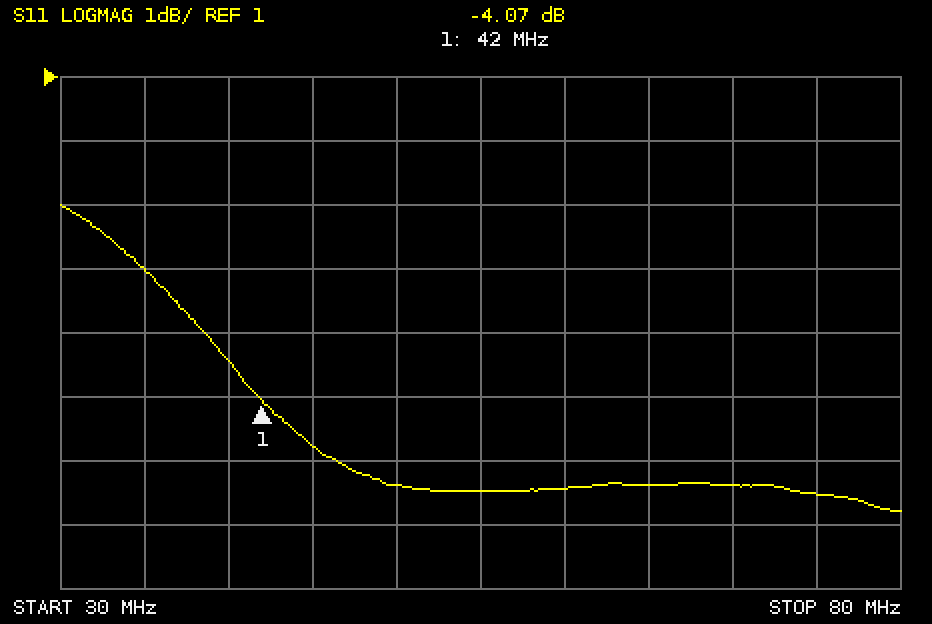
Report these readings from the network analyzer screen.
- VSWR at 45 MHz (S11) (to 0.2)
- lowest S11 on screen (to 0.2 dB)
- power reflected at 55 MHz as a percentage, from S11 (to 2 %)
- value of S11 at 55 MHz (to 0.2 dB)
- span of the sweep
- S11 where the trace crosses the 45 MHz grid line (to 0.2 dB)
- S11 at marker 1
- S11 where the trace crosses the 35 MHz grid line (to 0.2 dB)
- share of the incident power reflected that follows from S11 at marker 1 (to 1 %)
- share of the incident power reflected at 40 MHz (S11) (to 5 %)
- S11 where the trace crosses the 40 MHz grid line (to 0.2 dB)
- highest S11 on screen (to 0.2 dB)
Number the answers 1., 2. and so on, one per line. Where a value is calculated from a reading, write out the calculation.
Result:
1. |Γ| = 10^(-4.8/20) = 0.5754; VSWR = (1 + 0.5754)/(1 − 0.5754) ≈ 3.71, so 3.8 to the nearest 0.2
2. -5.8 dB
3. 10^(-5.4/10) ≈ 28.8 %, so 28 % to the nearest 2 %
4. -5.4 dB
5. 50 MHz
6. -4.8 dB
7. -4.07 dB
8. -2.0 dB
9. 10^(-4.07/10) ≈ 39 %
10. 10^(-3.4/10) ≈ 45.7 %, so 45 % to the nearest 5 %
11. -3.4 dB
12. -1.0 dB
